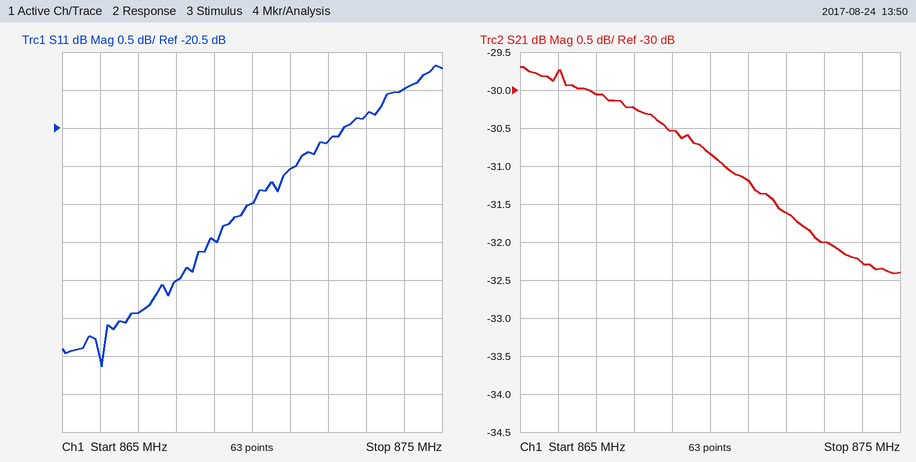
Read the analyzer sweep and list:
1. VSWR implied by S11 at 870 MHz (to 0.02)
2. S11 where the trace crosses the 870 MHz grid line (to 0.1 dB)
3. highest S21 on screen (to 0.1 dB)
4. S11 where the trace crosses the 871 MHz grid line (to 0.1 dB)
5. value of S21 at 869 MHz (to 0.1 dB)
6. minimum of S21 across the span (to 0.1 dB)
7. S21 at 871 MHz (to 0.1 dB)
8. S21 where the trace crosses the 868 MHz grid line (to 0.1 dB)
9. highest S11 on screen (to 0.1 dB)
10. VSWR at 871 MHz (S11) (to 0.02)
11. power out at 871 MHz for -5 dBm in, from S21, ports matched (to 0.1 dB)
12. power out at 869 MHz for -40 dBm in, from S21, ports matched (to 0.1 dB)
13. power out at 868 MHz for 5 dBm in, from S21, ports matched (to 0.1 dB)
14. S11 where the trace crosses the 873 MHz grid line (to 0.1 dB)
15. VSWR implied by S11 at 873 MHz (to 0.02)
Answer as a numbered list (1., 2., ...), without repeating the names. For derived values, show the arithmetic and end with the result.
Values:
1. |Γ| = 10^(-21.5/20) = 0.0841; VSWR = (1 + 0.0841)/(1 − 0.0841) ≈ 1.18
2. -21.5 dB
3. -29.7 dB
4. -21.0 dB
5. -30.5 dB
6. -32.4 dB
7. -31.2 dB
8. -30.2 dB
9. -19.7 dB
10. |Γ| = 10^(-21/20) = 0.0891; VSWR = (1 + 0.0891)/(1 − 0.0891) ≈ 1.20
11. -5 dBm + (-31.2 dB) = -36.2 dBm
12. -40 dBm + (-30.5 dB) = -70.5 dBm
13. 5 dBm + (-30.2 dB) = -25.2 dBm
14. -20.3 dB
15. |Γ| = 10^(-20.3/20) = 0.0966; VSWR = (1 + 0.0966)/(1 − 0.0966) ≈ 1.21, so 1.22 to the nearest 0.02
